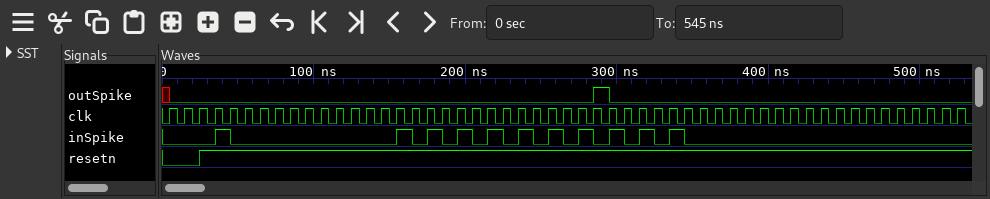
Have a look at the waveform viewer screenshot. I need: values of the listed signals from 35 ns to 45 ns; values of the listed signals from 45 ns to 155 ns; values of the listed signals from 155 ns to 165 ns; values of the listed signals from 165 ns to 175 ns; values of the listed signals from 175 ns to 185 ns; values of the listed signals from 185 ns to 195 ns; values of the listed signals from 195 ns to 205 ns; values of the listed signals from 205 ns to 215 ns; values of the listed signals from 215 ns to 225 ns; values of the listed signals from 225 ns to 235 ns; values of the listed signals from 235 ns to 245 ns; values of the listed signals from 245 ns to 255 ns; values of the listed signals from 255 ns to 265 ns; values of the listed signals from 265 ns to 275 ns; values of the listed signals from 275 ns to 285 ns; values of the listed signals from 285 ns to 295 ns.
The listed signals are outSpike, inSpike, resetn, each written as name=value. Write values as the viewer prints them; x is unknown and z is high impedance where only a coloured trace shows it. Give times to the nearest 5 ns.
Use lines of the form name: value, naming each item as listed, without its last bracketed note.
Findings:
values of the listed signals from 35 ns to 45 ns: outSpike=0, inSpike=1, resetn=1
values of the listed signals from 45 ns to 155 ns: outSpike=0, inSpike=0, resetn=1
values of the listed signals from 155 ns to 165 ns: outSpike=0, inSpike=1, resetn=1
values of the listed signals from 165 ns to 175 ns: outSpike=0, inSpike=0, resetn=1
values of the listed signals from 175 ns to 185 ns: outSpike=0, inSpike=1, resetn=1
values of the listed signals from 185 ns to 195 ns: outSpike=0, inSpike=0, resetn=1
values of the listed signals from 195 ns to 205 ns: outSpike=0, inSpike=1, resetn=1
values of the listed signals from 205 ns to 215 ns: outSpike=0, inSpike=0, resetn=1
values of the listed signals from 215 ns to 225 ns: outSpike=0, inSpike=1, resetn=1
values of the listed signals from 225 ns to 235 ns: outSpike=0, inSpike=0, resetn=1
values of the listed signals from 235 ns to 245 ns: outSpike=0, inSpike=1, resetn=1
values of the listed signals from 245 ns to 255 ns: outSpike=0, inSpike=0, resetn=1
values of the listed signals from 255 ns to 265 ns: outSpike=0, inSpike=1, resetn=1
values of the listed signals from 265 ns to 275 ns: outSpike=0, inSpike=0, resetn=1
values of the listed signals from 275 ns to 285 ns: outSpike=0, inSpike=1, resetn=1
values of the listed signals from 285 ns to 295 ns: outSpike=1, inSpike=0, resetn=1
